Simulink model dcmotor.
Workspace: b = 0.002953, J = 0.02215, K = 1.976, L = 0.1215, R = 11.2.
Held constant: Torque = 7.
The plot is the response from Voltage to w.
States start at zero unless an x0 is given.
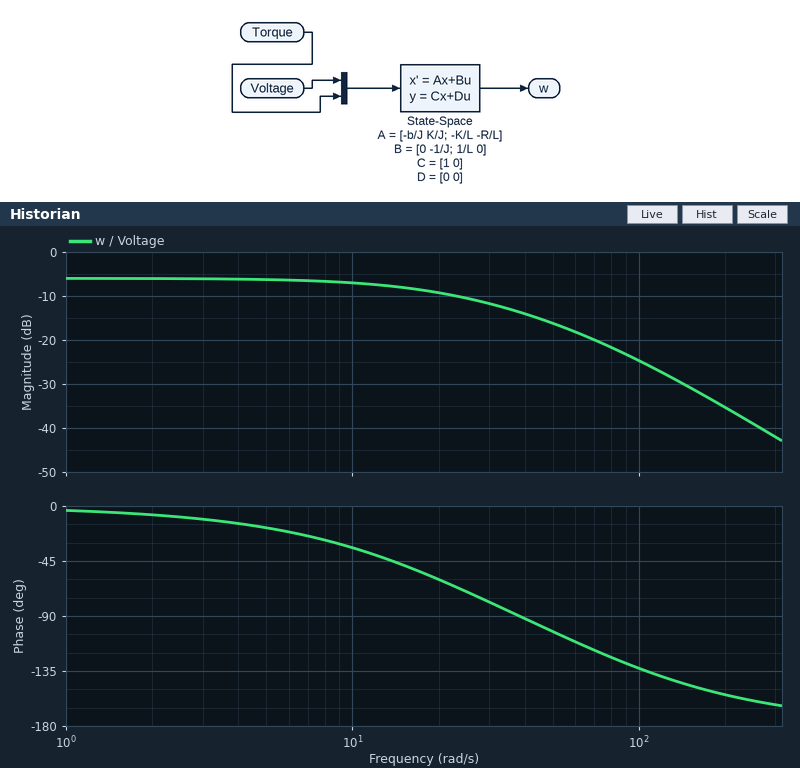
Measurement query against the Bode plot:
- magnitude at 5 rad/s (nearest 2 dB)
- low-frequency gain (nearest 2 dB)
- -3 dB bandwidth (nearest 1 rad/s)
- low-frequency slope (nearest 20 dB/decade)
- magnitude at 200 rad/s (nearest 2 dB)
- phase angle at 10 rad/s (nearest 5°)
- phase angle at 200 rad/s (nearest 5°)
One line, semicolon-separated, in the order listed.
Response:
-6 dB; -6 dB; 19 rad/s; 0 dB/decade; -36 dB; -35°; -155°
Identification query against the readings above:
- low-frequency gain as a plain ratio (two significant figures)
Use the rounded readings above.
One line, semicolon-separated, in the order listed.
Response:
0.50
